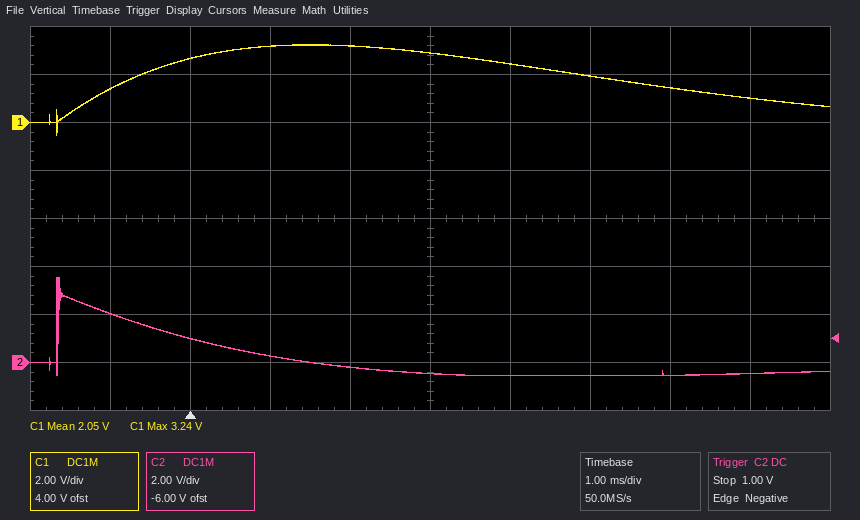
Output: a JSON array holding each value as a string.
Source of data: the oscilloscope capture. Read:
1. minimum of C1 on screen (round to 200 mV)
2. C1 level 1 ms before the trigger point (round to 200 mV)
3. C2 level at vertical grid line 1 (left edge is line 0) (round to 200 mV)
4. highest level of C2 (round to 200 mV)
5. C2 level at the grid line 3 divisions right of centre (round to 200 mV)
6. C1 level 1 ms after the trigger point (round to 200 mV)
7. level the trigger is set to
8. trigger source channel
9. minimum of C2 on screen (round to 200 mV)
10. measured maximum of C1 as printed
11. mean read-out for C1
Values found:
["-600 mV", "1.4 V", "2.0 V", "3.6 V", "-600 mV", "3.2 V", "1.00 V", "C2", "-600 mV", "3.24 V", "2.05 V"]
